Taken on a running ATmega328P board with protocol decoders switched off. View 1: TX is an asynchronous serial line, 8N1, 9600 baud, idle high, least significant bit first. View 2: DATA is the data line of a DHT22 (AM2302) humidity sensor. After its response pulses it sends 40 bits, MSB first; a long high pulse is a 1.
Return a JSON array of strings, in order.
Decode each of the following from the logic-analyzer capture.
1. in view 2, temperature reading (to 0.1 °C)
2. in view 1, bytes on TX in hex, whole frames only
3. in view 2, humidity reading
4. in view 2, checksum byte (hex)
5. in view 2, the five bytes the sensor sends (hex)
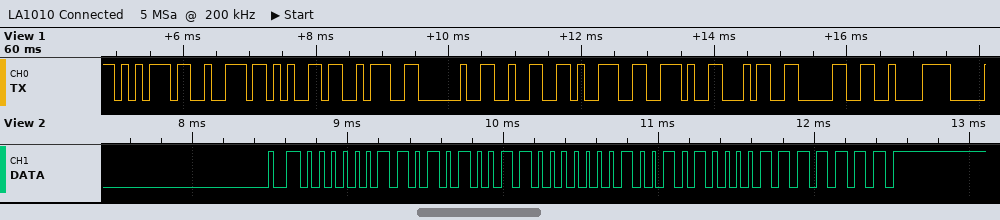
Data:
["29.6 °C", "75 72 65 3A 20 32 39 2E 34 30 C2", "85.1 %", "0x7F", "03 53 01 28 7F"]
